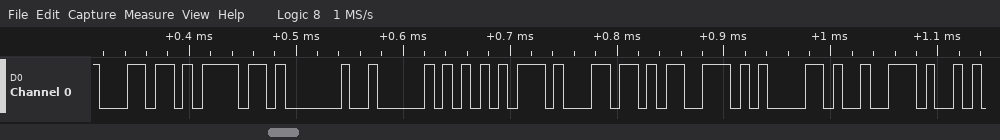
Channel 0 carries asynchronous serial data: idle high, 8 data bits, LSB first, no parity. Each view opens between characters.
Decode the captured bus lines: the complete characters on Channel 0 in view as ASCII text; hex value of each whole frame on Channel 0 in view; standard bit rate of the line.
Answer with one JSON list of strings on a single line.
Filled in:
["\"lo Pulsar\"", "6C, 6F, 20, 50, 75, 6C, 73, 61, 72", "115200 baud"]
